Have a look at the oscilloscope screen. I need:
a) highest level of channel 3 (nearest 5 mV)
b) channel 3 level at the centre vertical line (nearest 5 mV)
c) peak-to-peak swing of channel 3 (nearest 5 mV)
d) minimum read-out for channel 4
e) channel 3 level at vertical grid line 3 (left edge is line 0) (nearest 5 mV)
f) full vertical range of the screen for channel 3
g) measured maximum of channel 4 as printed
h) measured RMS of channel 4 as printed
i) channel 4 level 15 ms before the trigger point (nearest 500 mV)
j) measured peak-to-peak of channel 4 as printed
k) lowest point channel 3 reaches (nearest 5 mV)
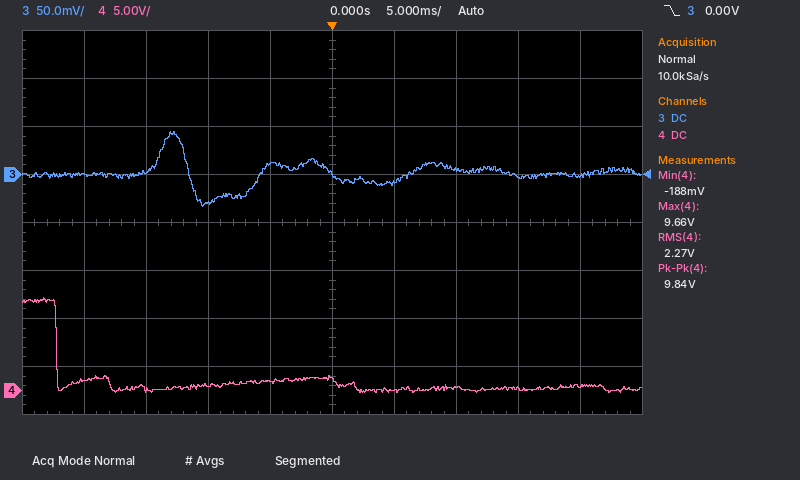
45 mV
0 mV
80 mV
-188 mV
-30 mV
400 mV
9.66 V
2.27 V
0.0 V
9.84 V
-35 mV
